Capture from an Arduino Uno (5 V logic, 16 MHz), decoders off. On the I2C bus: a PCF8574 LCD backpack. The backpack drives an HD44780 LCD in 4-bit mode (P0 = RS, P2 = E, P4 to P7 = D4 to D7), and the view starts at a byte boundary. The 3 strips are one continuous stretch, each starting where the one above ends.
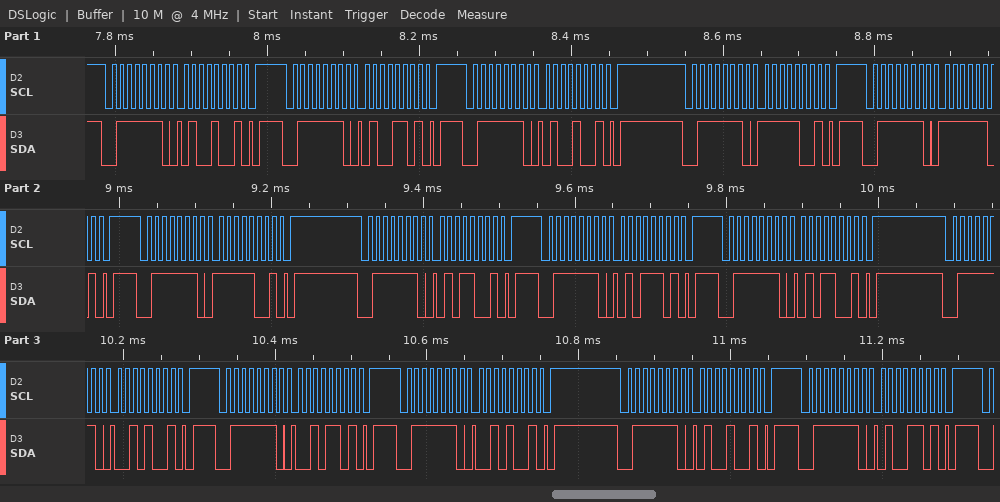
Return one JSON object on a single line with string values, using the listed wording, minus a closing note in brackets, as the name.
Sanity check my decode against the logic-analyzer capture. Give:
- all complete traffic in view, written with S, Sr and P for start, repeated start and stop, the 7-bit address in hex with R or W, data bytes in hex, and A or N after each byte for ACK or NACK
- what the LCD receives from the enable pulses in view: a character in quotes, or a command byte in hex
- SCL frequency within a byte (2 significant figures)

{"all complete traffic in view, written with S, Sr and P for start, repeated start and stop, the 7-bit address in hex with R or W, data bytes in hex, and A or N after each byte for ACK or NACK": "S 3FW A 49 A P S 3FW A 4D A P S 3FW A 49 A P S 3FW A F9 A P S 3FW A FD A P S 3FW A F9 A P S 3FW A 59 A P S 3FW A 5D A P S 3FW A 59 A P S 3FW A 29 A P S 3FW A 2D A P S 3FW A 29 A P S 3FW A 49 A P S 3FW A 4D A P", "what the LCD receives from the enable pulses in view: a character in quotes, or a command byte in hex": "'O' 'R'", "SCL frequency within a byte": "100 kHz"}
